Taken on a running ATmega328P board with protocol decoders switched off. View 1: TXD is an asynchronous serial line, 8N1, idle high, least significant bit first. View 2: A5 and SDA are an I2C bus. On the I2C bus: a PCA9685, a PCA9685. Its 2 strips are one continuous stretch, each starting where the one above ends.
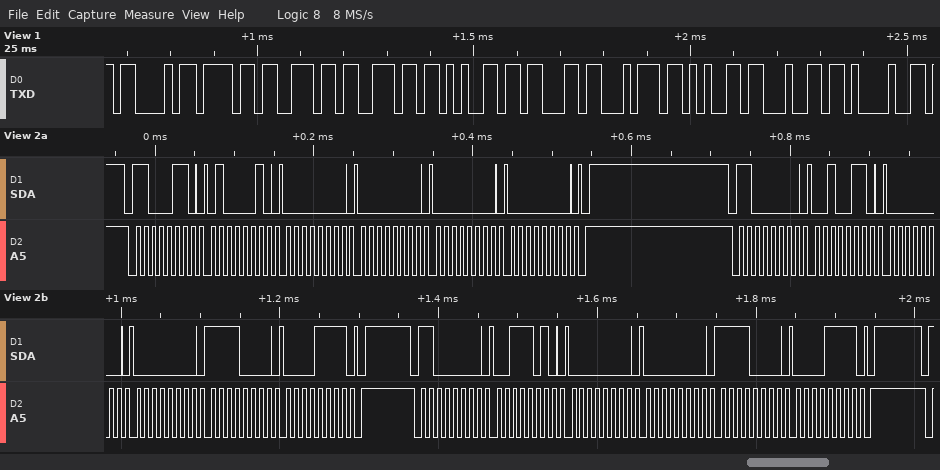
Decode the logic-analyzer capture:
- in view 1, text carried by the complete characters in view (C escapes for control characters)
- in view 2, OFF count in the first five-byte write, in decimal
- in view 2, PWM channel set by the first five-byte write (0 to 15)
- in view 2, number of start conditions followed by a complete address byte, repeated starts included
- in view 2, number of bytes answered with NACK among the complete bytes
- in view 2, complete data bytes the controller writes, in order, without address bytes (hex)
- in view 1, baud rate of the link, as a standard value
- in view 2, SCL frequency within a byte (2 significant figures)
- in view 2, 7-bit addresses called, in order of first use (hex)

"Connected!"
0
15
3
0
42 00 00 00 00 26 00 00 F0 0F 3A 00 00 F0 0F
57600 baud
100 kHz
0x63 0x60
